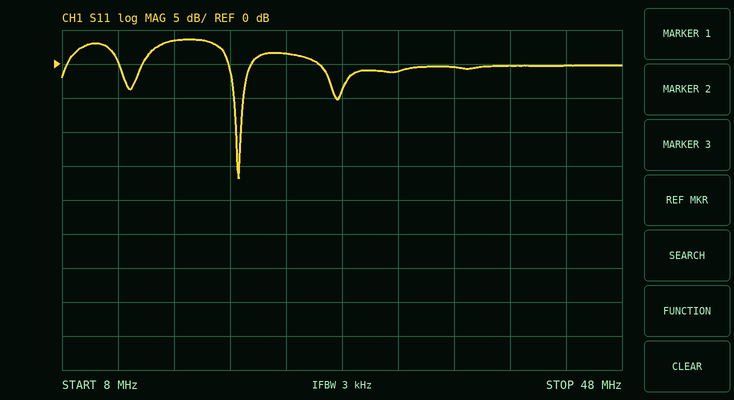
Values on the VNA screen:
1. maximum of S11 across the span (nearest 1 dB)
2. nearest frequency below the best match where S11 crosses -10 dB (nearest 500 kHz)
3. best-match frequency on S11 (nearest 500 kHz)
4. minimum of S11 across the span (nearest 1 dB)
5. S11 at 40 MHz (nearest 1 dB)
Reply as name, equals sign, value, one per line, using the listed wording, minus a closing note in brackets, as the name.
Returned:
maximum of S11 across the span = 4 dB
nearest frequency below the best match where S11 crosses -10 dB = 20.5 MHz
best-match frequency on S11 = 20.5 MHz
minimum of S11 across the span = -17 dB
S11 at 40 MHz = 0 dB
